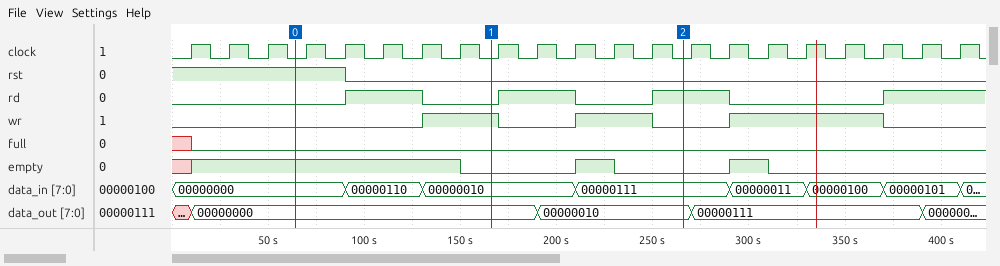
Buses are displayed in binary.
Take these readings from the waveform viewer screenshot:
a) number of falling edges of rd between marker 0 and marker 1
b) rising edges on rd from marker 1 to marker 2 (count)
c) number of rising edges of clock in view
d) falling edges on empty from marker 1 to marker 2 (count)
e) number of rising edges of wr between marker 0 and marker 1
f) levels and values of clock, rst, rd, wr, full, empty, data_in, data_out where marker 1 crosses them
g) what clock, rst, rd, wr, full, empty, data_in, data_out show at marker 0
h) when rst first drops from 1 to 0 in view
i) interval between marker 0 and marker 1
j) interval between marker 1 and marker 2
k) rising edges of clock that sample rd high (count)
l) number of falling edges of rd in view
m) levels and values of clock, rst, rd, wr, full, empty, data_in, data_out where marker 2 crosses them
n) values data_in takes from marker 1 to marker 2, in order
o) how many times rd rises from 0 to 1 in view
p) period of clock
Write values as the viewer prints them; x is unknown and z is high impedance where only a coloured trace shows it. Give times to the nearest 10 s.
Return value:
1
2
21
1
1
clock=0, rst=0, rd=0, wr=1, full=0, empty=0, data_in=00000010, data_out=00000000
clock=0, rst=1, rd=0, wr=0, full=0, empty=1, data_in=00000000, data_out=00000000
90 s
100 s
100 s
8
3
clock=0, rst=0, rd=1, wr=0, full=0, empty=0, data_in=00000111, data_out=00000010
00000010, 00000111
4
20 s
